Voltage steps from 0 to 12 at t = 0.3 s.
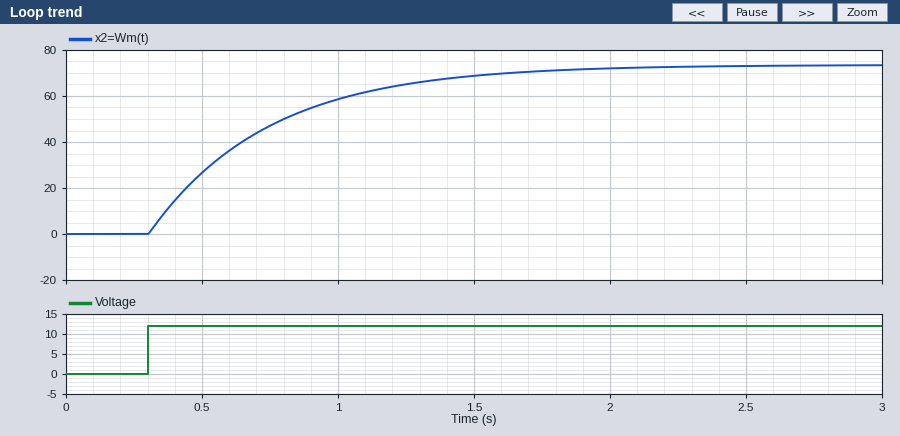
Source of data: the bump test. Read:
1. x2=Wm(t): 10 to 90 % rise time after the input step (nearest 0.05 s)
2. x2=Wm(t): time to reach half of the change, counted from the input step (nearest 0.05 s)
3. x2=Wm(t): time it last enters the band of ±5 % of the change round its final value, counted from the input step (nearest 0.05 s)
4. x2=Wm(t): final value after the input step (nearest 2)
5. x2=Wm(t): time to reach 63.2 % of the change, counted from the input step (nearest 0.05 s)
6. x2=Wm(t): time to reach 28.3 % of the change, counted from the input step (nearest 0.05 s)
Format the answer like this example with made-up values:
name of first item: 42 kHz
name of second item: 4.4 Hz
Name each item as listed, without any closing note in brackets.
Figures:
x2=Wm(t): 10 to 90 % rise time after the input step: 0.95 s
x2=Wm(t): time to reach half of the change, counted from the input step: 0.30 s
x2=Wm(t): time it last enters the band of ±5 % of the change round its final value, counted from the input step: 1.30 s
x2=Wm(t): final value after the input step: 74
x2=Wm(t): time to reach 63.2 % of the change, counted from the input step: 0.45 s
x2=Wm(t): time to reach 28.3 % of the change, counted from the input step: 0.15 s
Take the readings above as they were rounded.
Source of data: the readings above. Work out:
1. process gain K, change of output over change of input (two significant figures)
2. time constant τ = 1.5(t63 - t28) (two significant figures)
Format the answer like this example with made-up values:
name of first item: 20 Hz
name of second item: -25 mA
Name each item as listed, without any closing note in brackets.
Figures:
process gain K, change of output over change of input: 6.2
time constant τ = 1.5(t63 - t28): 0.45 s
